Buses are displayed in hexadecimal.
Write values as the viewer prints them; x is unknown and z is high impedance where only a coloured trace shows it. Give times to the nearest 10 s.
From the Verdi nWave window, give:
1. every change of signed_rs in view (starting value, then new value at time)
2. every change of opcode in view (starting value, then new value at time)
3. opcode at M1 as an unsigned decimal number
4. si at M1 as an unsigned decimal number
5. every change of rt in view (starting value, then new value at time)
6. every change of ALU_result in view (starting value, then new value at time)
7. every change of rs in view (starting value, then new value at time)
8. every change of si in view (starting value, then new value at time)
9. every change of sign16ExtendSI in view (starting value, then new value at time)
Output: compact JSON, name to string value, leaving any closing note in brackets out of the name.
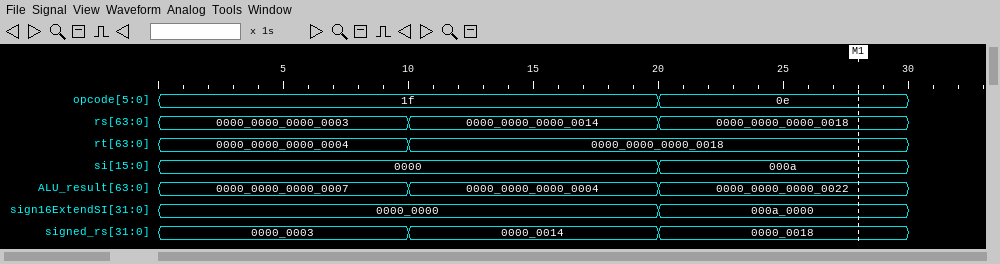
{"every change of signed_rs in view": "0000_0003, 0000_0014 at 10 s, 0000_0018 at 20 s", "every change of opcode in view": "1f, 0e at 20 s", "opcode at M1 as an unsigned decimal number": "14", "si at M1 as an unsigned decimal number": "10", "every change of rt in view": "0000_0000_0000_0004, 0000_0000_0000_0018 at 10 s", "every change of ALU_result in view": "0000_0000_0000_0007, 0000_0000_0000_0004 at 10 s, 0000_0000_0000_0022 at 20 s", "every change of rs in view": "0000_0000_0000_0003, 0000_0000_0000_0014 at 10 s, 0000_0000_0000_0018 at 20 s", "every change of si in view": "0000, 000a at 20 s", "every change of sign16ExtendSI in view": "0000_0000, 000a_0000 at 20 s"}
